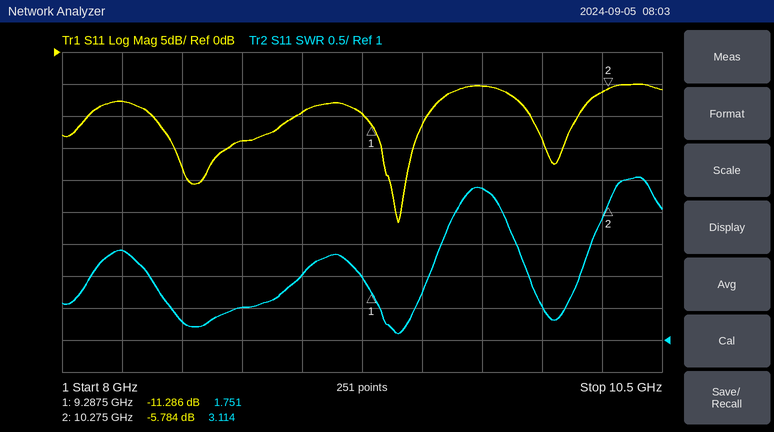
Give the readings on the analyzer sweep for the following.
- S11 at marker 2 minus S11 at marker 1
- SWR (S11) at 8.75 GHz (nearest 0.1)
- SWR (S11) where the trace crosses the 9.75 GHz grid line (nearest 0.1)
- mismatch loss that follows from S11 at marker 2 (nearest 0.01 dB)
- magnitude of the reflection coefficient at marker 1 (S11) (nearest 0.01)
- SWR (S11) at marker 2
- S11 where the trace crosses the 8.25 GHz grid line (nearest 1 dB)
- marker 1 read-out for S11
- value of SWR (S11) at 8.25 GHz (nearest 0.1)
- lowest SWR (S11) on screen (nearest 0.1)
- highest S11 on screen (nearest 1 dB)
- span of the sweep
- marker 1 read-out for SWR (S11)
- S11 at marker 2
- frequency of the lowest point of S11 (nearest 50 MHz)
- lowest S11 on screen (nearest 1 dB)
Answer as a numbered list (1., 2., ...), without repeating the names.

1. 5.502 dB
2. 1.5
3. 3.4
4. 1.33 dB
5. 0.27
6. 3.114
7. -8 dB
8. -11.286 dB
9. 2.4
10. 1.1
11. -5 dB
12. 2.5 GHz
13. 1.751
14. -5.784 dB
15. 9.40 GHz
16. -27 dB
